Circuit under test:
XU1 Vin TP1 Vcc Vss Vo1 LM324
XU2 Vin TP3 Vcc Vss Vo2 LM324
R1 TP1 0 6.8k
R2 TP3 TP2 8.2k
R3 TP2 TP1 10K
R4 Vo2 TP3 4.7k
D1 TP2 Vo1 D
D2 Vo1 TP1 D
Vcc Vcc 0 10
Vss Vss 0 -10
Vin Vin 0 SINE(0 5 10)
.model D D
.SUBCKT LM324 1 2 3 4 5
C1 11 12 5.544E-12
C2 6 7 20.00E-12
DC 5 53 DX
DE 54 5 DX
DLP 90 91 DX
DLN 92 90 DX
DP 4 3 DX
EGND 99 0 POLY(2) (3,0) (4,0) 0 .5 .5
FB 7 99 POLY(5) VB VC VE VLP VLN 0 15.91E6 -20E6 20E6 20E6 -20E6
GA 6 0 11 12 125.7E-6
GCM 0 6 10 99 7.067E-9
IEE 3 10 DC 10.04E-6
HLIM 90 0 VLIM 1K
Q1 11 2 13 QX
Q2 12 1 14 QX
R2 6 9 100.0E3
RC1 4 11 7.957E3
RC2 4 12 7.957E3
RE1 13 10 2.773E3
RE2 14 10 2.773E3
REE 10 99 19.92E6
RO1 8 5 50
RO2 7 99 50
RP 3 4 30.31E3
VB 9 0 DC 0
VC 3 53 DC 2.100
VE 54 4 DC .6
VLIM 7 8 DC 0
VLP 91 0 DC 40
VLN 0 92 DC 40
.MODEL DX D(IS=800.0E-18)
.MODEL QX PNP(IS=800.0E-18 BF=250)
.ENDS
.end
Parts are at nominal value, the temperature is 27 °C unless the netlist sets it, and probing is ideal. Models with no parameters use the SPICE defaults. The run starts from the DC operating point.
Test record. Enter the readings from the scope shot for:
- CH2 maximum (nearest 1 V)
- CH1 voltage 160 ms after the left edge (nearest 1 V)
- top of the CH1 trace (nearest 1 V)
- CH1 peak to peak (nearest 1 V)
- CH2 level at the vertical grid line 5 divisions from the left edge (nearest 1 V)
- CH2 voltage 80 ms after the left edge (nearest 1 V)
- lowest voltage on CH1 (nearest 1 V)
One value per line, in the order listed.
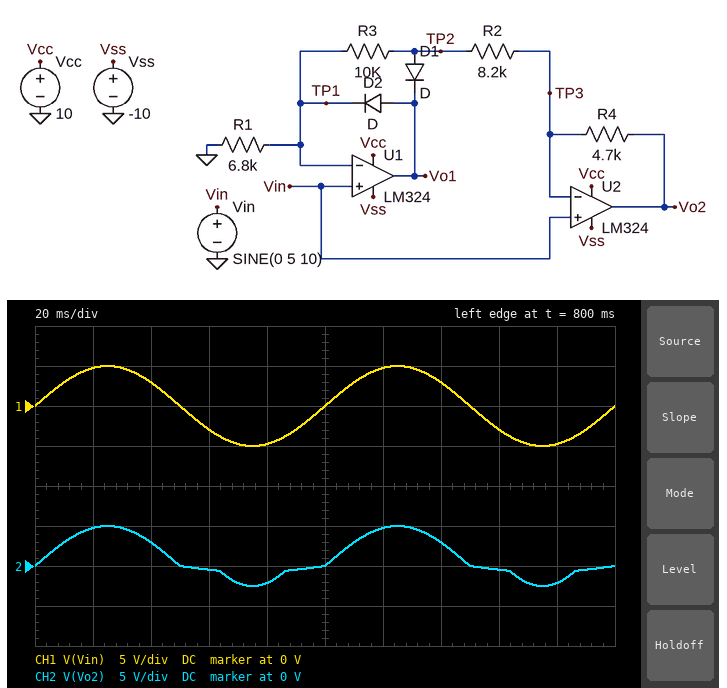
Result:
5 V
-3 V
5 V
10 V
0 V
-2 V
-5 V
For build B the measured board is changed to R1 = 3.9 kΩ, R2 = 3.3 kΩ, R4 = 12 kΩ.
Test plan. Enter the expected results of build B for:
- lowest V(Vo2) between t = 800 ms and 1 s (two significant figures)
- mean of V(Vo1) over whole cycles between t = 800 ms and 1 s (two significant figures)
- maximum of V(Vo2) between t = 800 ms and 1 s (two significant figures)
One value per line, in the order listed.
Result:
-17 mV
-2.3 V
8.5 V
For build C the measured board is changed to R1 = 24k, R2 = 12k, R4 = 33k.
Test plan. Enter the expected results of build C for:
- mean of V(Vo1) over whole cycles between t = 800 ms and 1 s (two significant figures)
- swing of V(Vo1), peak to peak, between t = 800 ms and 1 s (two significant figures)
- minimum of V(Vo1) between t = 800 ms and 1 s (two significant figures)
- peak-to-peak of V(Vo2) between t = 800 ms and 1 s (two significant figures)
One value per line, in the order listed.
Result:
-670 mV
13 V
-7.7 V
5.0 V
